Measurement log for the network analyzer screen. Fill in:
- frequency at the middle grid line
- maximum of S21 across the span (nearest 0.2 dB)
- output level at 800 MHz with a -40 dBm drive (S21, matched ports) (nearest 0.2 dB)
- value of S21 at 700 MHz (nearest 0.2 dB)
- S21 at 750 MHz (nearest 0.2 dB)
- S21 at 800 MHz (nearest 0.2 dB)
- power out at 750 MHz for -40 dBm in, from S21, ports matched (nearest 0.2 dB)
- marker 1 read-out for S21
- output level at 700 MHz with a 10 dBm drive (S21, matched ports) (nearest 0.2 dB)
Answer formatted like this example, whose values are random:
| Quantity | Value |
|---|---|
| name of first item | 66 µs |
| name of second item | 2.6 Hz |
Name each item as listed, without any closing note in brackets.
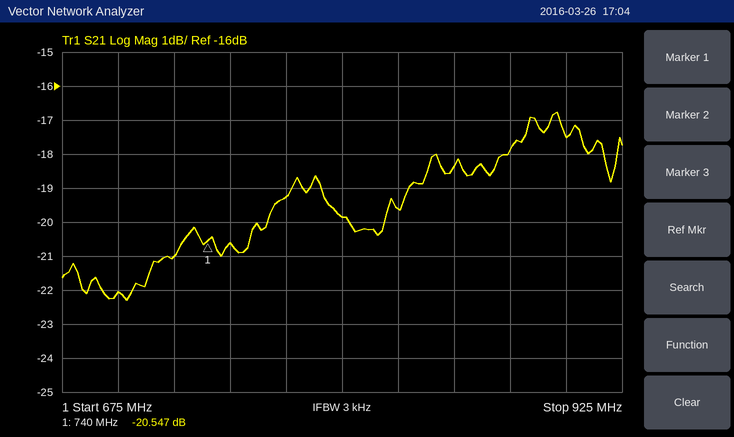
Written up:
| Quantity | Value |
|---|---|
| frequency at the middle grid line | 800 MHz |
| maximum of S21 across the span | -16.8 dB |
| output level at 800 MHz with a -40 dBm drive (S21, matched ports) | -59.8 dBm |
| value of S21 at 700 MHz | -22.0 dB |
| S21 at 750 MHz | -20.6 dB |
| S21 at 800 MHz | -19.8 dB |
| power out at 750 MHz for -40 dBm in, from S21, ports matched | -60.6 dBm |
| marker 1 read-out for S21 | -20.547 dB |
| output level at 700 MHz with a 10 dBm drive (S21, matched ports) | -12.0 dBm |
